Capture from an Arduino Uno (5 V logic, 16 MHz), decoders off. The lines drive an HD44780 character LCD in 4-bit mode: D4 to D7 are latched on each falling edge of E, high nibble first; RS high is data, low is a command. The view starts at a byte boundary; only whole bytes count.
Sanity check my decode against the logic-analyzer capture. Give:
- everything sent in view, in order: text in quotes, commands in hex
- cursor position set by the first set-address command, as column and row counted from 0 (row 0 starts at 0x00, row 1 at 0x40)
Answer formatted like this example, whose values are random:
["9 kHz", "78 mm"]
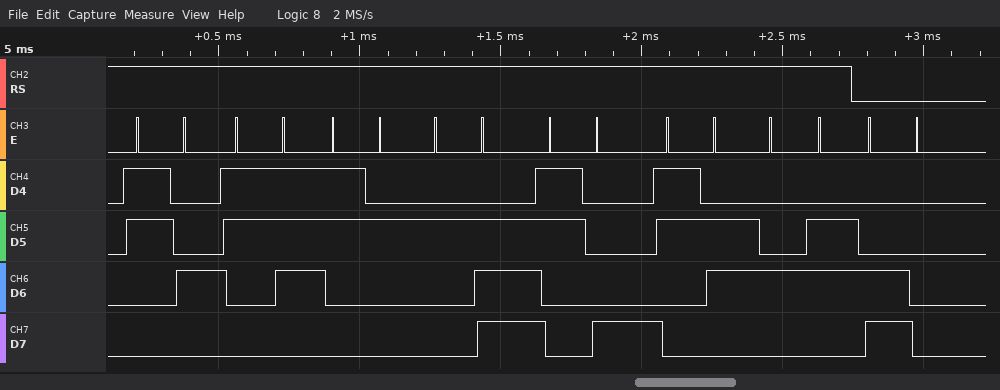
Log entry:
["\"472.86F\" 0xC0", "column 0, row 1"]
